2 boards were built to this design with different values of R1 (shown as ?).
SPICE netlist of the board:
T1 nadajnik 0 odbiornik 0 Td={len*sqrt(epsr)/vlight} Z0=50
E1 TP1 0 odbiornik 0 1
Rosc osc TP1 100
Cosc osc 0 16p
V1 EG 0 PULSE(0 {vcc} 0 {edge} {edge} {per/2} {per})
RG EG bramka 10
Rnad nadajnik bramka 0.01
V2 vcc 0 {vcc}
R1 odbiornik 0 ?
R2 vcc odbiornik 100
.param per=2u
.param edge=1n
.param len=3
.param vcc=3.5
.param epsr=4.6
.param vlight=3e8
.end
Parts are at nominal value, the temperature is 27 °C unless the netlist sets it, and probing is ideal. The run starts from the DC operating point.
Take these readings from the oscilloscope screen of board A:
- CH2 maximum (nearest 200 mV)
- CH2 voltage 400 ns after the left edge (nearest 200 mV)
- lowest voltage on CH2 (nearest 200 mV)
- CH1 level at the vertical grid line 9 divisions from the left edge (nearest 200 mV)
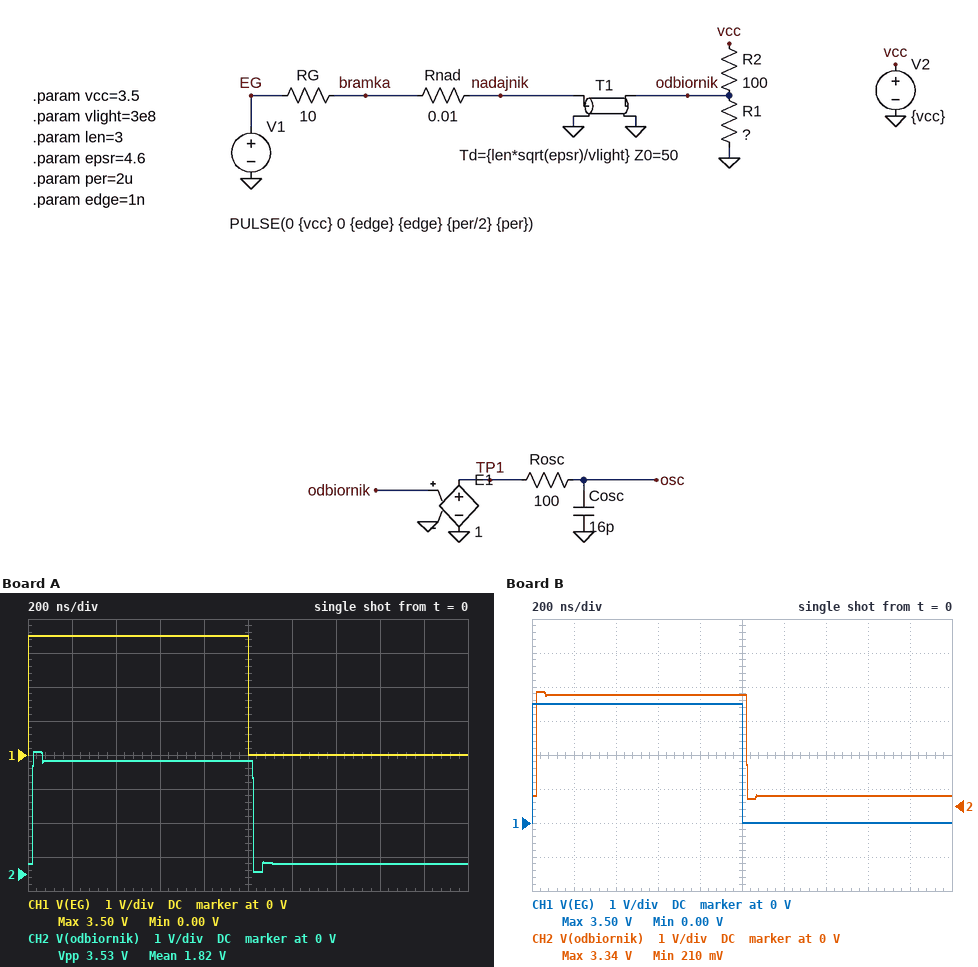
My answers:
3.6 V
3.4 V
0 V
0 V
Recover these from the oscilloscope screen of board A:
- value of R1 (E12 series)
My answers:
180 Ω
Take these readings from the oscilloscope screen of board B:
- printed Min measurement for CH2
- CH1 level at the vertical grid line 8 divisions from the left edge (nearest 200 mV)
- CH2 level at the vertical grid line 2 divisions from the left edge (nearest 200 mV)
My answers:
210 mV
0 V
3.2 V
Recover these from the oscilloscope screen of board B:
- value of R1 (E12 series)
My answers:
120 Ω
